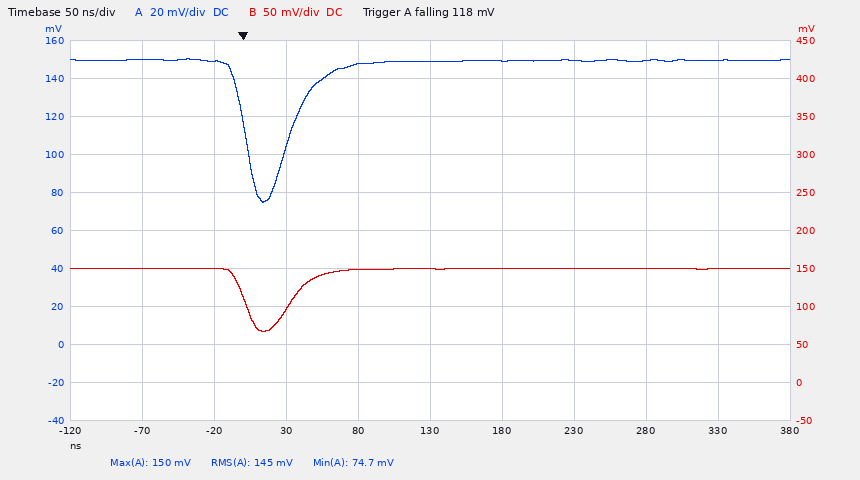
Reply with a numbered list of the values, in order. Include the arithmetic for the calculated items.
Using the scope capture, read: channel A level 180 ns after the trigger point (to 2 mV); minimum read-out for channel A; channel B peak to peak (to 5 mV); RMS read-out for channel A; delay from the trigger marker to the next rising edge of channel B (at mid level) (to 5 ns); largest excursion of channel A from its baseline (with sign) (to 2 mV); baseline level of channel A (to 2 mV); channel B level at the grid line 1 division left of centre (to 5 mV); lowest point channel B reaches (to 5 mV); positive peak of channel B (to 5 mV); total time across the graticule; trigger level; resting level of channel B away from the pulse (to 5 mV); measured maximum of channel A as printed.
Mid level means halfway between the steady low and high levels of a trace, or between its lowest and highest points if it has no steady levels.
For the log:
1. 150 mV
2. 74.7 mV
3. 150 mV − (65 mV) = 85 mV
4. 145 mV
5. 35 ns
6. -74 mV
7. 150 mV
8. 150 mV
9. 65 mV
10. 150 mV
11. 500 ns
12. 118 mV
13. 150 mV
14. 150 mV
